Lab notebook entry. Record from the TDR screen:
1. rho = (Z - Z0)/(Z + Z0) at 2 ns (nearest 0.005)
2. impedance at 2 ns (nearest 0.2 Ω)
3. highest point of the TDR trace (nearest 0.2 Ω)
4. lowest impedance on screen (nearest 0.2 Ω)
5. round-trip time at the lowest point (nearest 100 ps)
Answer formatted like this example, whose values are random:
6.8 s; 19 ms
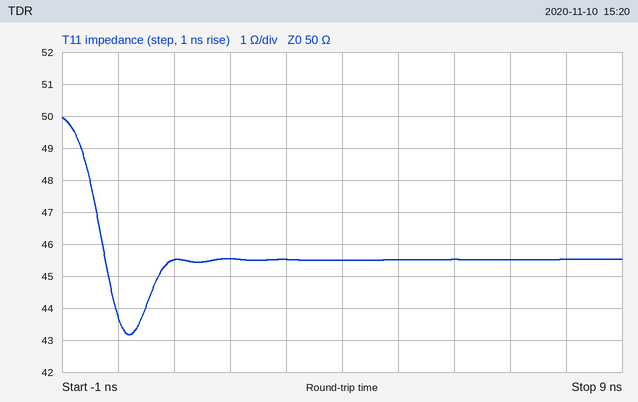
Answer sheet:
-0.045; 45.6 Ω; 50.0 Ω; 43.2 Ω; 200 ps
